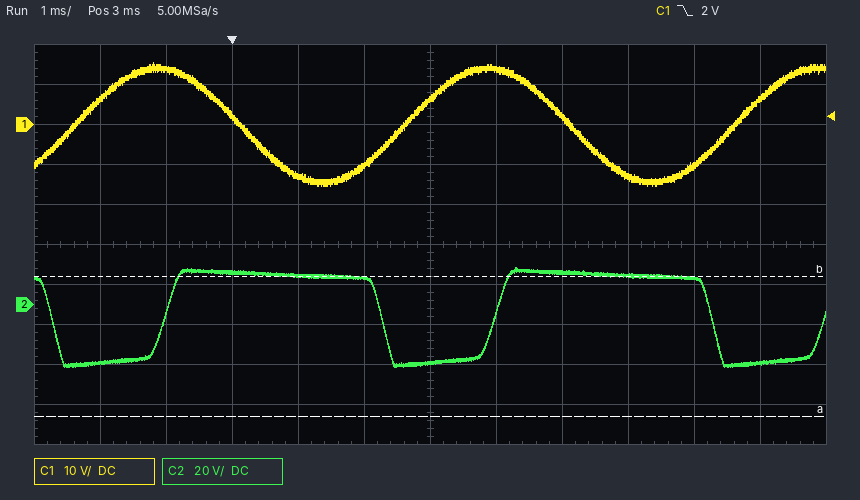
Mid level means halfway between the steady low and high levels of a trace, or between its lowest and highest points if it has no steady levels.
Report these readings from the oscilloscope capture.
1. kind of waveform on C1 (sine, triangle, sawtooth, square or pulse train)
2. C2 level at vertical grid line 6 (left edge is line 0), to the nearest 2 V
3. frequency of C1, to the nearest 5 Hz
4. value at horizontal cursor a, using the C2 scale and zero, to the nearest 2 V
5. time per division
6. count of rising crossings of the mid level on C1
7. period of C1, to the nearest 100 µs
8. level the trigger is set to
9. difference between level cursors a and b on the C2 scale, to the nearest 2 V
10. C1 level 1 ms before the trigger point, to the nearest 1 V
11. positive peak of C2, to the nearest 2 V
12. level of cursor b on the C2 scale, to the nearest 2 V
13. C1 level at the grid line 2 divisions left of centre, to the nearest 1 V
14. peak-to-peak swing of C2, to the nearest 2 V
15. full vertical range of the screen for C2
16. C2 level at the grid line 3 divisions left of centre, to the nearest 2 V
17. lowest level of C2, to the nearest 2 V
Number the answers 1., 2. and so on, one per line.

1. sine
2. -30 V
3. 200 Hz
4. -56 V
5. 1 ms
6. 3
7. 5.0 ms
8. 2 V
9. 70 V
10. 14 V
11. 18 V
12. 14 V
13. -13 V
14. 50 V
15. 200 V
16. 16 V
17. -32 V
